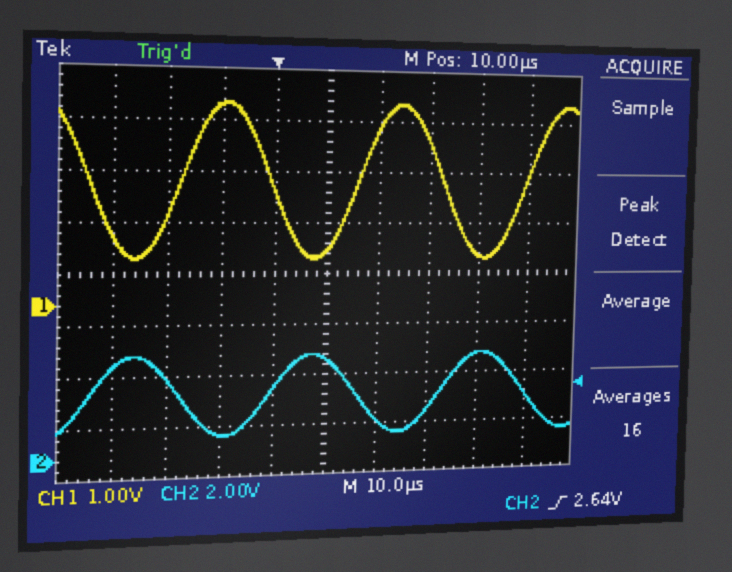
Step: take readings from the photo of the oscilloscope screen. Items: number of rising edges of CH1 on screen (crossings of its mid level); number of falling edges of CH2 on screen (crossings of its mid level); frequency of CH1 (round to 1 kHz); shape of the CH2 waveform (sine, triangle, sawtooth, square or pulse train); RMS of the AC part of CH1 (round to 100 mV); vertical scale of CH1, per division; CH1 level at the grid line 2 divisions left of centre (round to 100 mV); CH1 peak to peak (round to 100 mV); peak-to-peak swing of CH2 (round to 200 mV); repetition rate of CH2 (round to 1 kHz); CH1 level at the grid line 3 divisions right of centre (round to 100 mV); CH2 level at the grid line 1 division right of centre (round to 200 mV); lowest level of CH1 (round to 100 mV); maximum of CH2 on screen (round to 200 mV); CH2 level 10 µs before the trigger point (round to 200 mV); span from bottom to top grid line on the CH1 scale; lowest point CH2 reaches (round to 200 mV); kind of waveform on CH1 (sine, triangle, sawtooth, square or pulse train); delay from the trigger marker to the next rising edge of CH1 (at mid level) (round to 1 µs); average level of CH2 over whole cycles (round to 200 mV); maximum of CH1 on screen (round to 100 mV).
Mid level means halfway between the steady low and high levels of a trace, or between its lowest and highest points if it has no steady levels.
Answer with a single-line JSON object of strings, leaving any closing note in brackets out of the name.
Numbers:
{"number of rising edges of CH1 on screen": "3", "number of falling edges of CH2 on screen": "3", "frequency of CH1": "30 kHz", "shape of the CH2 waveform": "sine", "RMS of the AC part of CH1": "1.1 V", "vertical scale of CH1, per division": "1 V", "CH1 level at the grid line 2 divisions left of centre": "3.9 V", "CH1 peak to peak": "3.1 V", "peak-to-peak swing of CH2": "3.2 V", "repetition rate of CH2": "30 kHz", "CH1 level at the grid line 3 divisions right of centre": "1.0 V", "CH2 level at the grid line 1 division right of centre": "1.4 V", "lowest level of CH1": "900 mV", "maximum of CH2 on screen": "4.0 V", "CH2 level 10 µs before the trigger point": "800 mV", "span from bottom to top grid line on the CH1 scale": "8 V", "lowest point CH2 reaches": "800 mV", "kind of waveform on CH1": "sine", "delay from the trigger marker to the next rising edge of CH1 (at mid level)": "16 µs", "average level of CH2 over whole cycles": "2.4 V", "maximum of CH1 on screen": "4.0 V"}
